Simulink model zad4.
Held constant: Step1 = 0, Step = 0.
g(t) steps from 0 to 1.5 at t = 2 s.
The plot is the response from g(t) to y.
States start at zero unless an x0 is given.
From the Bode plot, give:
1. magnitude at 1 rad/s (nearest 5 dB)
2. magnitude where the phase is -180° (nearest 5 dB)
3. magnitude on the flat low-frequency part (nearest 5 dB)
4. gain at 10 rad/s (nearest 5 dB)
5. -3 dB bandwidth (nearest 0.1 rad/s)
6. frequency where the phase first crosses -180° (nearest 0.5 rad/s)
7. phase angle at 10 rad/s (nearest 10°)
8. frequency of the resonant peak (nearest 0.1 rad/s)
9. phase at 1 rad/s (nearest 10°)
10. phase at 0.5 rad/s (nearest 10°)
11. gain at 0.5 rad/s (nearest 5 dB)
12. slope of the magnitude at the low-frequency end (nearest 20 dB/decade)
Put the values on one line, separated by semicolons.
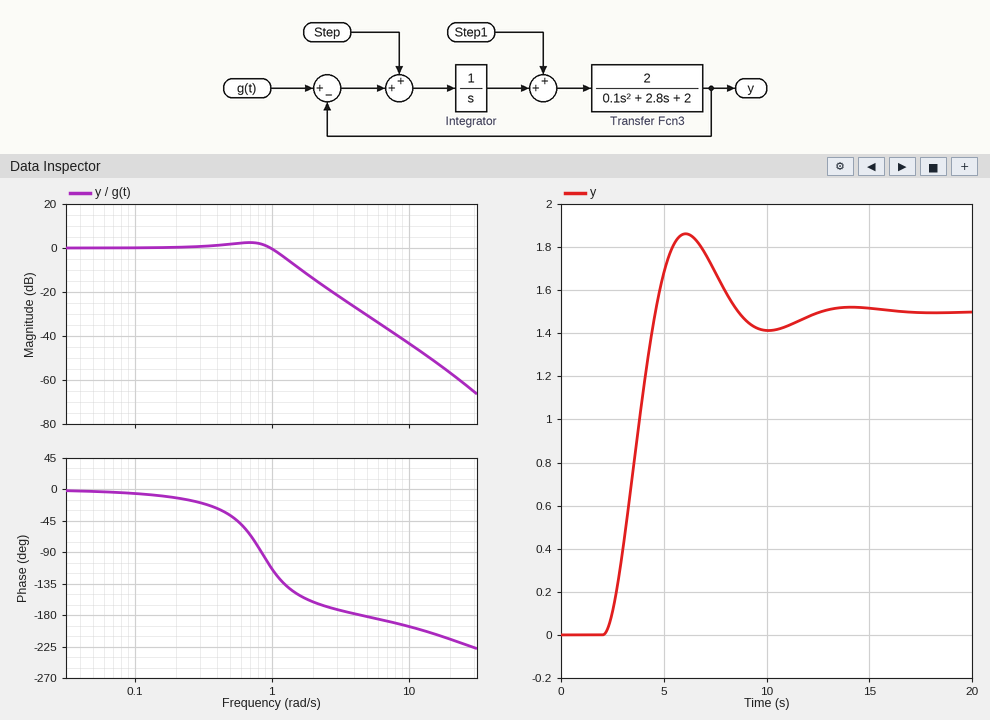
0 dB; -30 dB; 0 dB; -45 dB; 1.2 rad/s; 4.5 rad/s; -200°; 0.7 rad/s; -110°; -40°; 0 dB; 0 dB/decade
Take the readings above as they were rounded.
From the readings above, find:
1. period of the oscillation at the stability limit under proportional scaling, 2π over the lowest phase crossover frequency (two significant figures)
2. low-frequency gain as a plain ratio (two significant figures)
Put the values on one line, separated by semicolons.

1.4 s; 1.0
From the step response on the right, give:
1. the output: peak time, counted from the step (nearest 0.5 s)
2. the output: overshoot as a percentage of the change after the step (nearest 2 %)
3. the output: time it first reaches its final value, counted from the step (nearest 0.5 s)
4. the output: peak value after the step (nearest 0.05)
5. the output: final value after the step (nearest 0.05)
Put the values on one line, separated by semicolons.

4.0 s; 24 %; 2.5 s; 1.85; 1.50
